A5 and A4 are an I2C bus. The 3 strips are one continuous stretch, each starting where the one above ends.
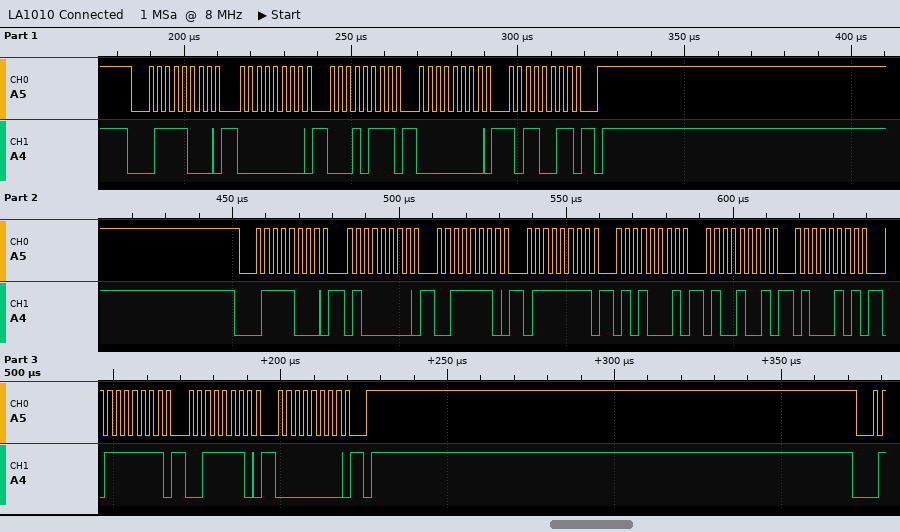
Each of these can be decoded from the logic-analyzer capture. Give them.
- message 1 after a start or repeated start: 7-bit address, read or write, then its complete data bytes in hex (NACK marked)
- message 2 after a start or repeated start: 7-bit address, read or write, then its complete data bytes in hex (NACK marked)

0x3C write: 00 17 00 B3
0x3C write: 40 3E 7F 51 49 45 7F 3E 00
